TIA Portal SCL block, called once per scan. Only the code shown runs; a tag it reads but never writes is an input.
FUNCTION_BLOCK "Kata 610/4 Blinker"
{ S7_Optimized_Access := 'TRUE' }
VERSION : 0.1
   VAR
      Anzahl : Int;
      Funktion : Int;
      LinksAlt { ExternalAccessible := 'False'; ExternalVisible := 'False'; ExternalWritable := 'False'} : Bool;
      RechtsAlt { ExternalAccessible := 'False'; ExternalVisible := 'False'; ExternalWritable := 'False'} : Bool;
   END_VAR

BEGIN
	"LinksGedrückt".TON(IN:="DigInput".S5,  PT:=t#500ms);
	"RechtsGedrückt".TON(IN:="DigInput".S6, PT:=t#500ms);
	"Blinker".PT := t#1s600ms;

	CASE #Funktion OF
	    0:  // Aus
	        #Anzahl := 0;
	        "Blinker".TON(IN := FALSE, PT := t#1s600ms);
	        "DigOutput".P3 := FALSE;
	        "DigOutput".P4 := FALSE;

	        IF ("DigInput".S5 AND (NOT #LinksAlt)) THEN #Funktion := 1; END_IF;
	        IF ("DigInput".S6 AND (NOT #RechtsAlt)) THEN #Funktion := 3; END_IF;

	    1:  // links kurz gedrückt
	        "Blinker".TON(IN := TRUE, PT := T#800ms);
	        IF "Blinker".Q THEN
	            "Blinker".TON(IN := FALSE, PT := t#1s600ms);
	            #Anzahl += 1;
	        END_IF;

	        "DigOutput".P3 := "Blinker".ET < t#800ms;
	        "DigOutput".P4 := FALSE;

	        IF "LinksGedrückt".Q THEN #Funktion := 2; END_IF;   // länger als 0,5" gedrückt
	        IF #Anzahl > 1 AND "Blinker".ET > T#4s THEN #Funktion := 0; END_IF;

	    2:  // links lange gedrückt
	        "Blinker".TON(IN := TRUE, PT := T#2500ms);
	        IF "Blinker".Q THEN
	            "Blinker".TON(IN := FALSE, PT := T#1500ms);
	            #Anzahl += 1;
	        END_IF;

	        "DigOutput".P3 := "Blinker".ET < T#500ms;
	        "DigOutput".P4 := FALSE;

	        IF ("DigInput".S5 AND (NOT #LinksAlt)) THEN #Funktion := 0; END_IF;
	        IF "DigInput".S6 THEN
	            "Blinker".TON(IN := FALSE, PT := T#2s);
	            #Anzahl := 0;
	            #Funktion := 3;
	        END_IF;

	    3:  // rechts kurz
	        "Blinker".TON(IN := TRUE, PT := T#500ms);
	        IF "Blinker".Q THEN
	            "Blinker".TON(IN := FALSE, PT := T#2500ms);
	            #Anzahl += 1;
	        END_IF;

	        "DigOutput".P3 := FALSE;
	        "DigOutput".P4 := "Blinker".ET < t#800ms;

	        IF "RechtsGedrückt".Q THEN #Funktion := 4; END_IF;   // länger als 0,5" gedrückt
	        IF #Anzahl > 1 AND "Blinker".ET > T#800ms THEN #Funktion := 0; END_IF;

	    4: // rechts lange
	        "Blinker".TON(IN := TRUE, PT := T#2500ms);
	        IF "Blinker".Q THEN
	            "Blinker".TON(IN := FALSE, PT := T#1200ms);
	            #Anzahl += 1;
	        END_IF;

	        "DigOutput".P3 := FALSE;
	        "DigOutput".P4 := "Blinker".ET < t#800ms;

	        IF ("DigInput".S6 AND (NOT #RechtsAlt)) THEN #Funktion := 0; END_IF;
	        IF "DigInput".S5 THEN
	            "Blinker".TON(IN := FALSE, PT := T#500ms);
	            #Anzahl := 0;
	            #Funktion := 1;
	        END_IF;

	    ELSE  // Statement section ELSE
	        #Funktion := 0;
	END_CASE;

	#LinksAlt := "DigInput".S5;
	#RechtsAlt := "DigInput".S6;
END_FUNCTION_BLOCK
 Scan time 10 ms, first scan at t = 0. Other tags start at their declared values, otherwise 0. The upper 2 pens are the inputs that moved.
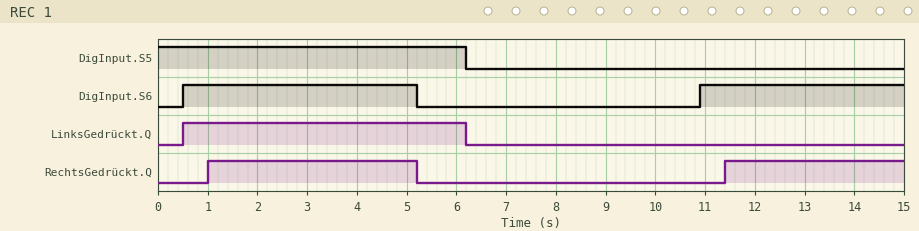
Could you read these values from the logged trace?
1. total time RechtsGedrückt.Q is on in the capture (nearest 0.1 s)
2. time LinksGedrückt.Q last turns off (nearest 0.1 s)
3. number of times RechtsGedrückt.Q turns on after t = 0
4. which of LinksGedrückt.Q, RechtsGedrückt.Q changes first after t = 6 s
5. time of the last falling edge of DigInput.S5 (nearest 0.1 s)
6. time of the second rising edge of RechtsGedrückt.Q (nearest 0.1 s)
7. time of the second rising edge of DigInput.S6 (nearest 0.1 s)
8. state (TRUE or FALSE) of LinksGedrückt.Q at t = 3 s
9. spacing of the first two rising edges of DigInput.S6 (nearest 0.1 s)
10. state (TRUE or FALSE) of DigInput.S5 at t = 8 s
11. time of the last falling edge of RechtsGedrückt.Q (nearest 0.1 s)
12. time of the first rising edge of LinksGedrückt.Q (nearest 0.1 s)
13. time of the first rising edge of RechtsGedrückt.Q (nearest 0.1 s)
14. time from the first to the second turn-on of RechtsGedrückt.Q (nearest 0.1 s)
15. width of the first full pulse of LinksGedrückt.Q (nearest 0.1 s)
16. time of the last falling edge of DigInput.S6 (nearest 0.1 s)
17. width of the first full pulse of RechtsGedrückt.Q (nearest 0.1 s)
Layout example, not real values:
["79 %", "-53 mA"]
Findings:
["7.8 s", "6.2 s", "2", "LinksGedrückt.Q", "6.2 s", "11.4 s", "10.9 s", "TRUE", "10.4 s", "FALSE", "5.2 s", "0.5 s", "1.0 s", "10.4 s", "5.7 s", "5.2 s", "4.2 s"]
